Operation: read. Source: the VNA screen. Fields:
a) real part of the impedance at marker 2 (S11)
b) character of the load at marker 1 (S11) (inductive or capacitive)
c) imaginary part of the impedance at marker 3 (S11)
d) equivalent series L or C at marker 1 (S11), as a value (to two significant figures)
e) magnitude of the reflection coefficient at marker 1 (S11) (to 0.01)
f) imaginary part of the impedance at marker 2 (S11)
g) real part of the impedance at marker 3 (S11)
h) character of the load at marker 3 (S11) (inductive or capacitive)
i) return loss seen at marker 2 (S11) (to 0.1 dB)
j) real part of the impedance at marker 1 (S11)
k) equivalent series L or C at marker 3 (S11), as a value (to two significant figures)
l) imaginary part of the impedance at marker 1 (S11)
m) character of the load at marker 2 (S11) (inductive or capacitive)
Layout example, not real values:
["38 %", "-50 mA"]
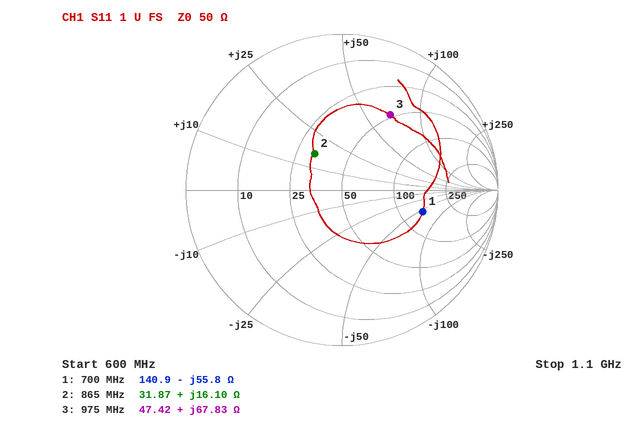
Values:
["31.87 Ω", "capacitive", "+67.83 Ω", "4.1 pF", "0.54", "+16.10 Ω", "47.42 Ω", "inductive", "10.7 dB", "140.9 Ω", "11 nH", "-55.8 Ω", "inductive"]
